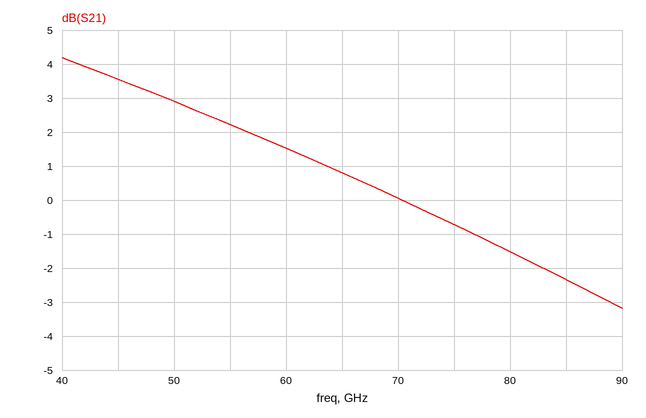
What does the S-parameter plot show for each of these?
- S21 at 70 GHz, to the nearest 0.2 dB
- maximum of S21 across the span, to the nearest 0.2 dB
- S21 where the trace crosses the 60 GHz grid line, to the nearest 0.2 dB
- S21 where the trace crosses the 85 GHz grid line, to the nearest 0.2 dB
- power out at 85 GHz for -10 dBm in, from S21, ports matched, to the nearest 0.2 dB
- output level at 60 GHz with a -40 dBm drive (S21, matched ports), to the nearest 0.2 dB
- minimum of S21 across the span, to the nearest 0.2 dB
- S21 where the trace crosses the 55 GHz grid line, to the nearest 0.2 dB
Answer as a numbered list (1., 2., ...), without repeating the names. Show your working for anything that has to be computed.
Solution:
1. 0.0 dB
2. 4.2 dB
3. 1.6 dB
4. -2.4 dB
5. -10 dBm + (-2.4 dB) = -12.4 dBm
6. -40 dBm + (1.6 dB) = -38.4 dBm
7. -3.2 dB
8. 2.2 dB
